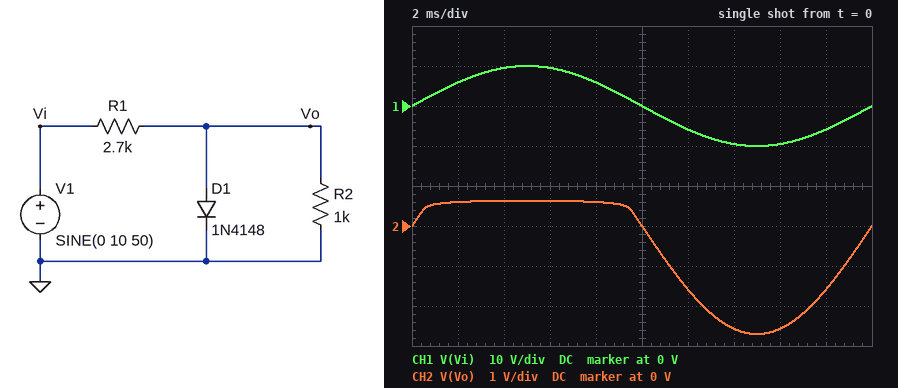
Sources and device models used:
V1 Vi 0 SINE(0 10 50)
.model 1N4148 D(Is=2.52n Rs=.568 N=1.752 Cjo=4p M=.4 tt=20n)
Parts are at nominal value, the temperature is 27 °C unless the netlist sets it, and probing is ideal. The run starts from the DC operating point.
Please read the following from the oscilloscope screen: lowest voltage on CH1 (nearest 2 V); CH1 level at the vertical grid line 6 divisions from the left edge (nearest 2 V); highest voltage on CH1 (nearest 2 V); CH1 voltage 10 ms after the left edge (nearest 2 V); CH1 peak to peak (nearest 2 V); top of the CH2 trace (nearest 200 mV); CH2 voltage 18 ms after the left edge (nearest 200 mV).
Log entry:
-10 V
-6 V
10 V
0 V
20 V
600 mV
-1.6 V
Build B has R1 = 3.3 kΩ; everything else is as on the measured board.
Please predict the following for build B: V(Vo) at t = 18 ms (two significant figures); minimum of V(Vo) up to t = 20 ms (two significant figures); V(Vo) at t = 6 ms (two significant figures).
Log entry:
-1.4 V
-2.3 V
620 mV
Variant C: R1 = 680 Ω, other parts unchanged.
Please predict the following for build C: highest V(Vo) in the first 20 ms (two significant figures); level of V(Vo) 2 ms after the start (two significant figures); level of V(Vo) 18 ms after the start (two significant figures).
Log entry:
710 mV
680 mV
-3.5 V
